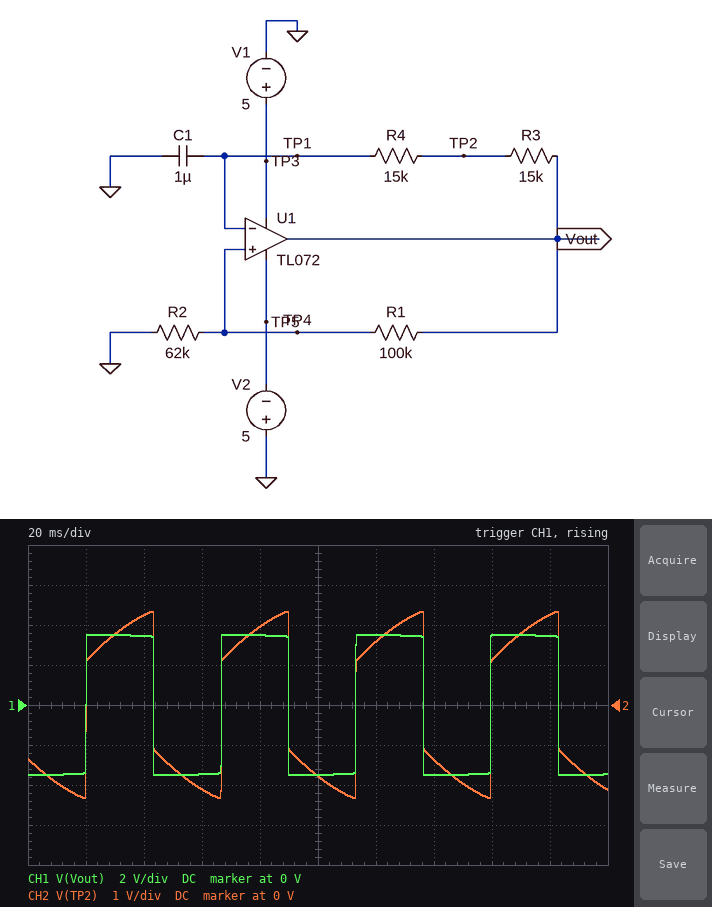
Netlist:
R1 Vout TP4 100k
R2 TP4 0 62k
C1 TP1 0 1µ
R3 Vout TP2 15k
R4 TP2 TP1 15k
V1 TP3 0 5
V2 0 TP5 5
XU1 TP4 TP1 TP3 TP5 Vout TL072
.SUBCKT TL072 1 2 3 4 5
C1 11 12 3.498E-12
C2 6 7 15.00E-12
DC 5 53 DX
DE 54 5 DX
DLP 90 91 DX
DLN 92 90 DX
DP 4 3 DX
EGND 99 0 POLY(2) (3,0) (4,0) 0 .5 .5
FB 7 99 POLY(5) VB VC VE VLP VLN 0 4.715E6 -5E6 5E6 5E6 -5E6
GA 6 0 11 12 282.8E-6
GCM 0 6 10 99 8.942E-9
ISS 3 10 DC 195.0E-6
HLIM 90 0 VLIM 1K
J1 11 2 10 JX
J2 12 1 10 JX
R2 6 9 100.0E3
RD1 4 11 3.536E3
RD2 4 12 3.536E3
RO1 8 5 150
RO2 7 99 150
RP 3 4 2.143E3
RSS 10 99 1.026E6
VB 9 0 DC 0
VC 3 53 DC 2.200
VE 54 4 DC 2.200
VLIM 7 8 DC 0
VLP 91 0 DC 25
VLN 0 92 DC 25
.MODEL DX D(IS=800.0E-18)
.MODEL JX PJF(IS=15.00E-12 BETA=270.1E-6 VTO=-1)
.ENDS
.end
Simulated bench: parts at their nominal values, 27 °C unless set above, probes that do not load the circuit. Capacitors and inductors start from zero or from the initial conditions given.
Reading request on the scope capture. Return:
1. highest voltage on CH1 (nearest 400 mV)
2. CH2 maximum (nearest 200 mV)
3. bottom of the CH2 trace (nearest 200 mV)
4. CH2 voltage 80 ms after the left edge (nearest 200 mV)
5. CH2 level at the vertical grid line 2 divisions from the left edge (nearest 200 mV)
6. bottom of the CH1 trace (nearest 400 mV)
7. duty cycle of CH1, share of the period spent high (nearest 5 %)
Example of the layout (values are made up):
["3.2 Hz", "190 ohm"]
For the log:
["3.6 V", "2.4 V", "-2.4 V", "2.0 V", "2.2 V", "-3.6 V", "50 %"]
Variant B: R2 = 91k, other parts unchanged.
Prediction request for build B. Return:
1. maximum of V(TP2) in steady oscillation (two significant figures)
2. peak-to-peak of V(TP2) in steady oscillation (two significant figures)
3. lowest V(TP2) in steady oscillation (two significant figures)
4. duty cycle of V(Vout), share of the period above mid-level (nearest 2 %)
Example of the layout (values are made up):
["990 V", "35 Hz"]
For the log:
["2.5 V", "5.0 V", "-2.5 V", "50 %"]
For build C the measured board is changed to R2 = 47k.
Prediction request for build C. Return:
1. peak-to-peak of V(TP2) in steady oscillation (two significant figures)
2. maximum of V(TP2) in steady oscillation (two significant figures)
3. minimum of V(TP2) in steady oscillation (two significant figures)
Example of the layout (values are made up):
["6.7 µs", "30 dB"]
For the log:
["4.5 V", "2.2 V", "-2.2 V"]
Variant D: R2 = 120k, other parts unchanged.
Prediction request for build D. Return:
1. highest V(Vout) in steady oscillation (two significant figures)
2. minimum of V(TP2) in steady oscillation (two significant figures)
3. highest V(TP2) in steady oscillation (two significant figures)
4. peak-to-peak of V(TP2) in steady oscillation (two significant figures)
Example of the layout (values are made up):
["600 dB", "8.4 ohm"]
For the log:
["3.5 V", "-2.6 V", "2.6 V", "5.2 V"]
